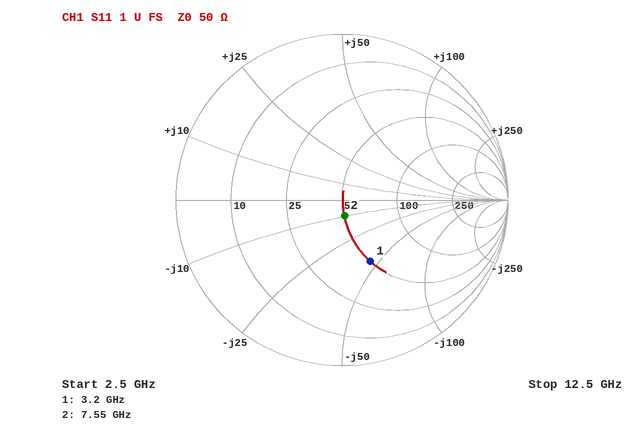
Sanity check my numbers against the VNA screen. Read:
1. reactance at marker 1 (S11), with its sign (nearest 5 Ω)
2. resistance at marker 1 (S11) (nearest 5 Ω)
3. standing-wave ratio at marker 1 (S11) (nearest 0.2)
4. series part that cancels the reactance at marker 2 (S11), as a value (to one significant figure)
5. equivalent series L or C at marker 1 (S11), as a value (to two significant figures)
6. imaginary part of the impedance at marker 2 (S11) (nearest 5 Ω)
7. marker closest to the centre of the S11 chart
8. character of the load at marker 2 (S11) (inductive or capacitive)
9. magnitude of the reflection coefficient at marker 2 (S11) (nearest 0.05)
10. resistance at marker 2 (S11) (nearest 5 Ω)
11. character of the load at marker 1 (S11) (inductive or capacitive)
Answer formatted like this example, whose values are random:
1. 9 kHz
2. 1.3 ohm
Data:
1. -45 Ω
2. 50 Ω
3. 2.4
4. 200 pH
5. 1.1 pF
6. -10 Ω
7. marker 2
8. capacitive
9. 0.10
10. 50 Ω
11. capacitive
